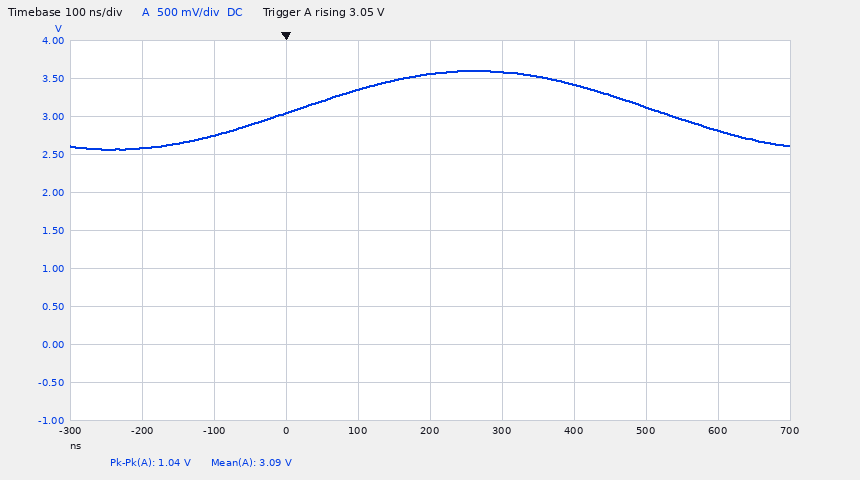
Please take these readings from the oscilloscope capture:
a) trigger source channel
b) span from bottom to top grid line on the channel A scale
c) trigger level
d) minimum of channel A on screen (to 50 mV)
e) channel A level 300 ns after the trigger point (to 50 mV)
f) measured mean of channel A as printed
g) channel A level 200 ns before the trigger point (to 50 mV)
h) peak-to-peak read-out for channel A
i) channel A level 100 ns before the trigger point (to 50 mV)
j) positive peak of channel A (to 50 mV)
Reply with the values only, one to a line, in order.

channel A
5 V
3.05 V
2.55 V
3.60 V
3.09 V
2.60 V
1.04 V
2.75 V
3.60 V
